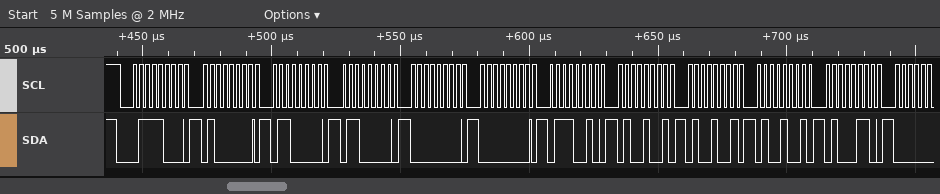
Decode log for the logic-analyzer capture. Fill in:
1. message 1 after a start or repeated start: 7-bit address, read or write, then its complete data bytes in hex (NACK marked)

0x3C write: 40 60 60 00 00 72 49 49 49 46
